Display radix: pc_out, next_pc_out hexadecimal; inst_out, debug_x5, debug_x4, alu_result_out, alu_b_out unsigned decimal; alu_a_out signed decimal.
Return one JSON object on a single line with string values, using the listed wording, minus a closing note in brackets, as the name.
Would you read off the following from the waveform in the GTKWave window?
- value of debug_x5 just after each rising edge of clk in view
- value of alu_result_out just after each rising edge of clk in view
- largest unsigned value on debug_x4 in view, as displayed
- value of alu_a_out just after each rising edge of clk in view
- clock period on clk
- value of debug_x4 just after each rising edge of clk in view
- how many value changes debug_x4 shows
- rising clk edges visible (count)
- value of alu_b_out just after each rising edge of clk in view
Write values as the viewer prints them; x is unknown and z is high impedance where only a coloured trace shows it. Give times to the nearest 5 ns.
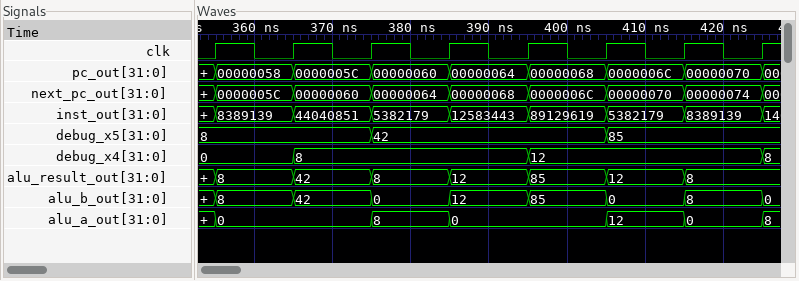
{"value of debug_x5 just after each rising edge of clk in view": "8, 8, 42, 42, 42, 85, 85, 85", "value of alu_result_out just after each rising edge of clk in view": "8, 42, 8, 12, 85, 12, 8, 8", "largest unsigned value on debug_x4 in view, as displayed": "12", "value of alu_a_out just after each rising edge of clk in view": "0, 0, 8, 0, 0, 12, 0, 8", "clock period on clk": "10 ns", "value of debug_x4 just after each rising edge of clk in view": "0, 8, 8, 8, 12, 12, 12, 8", "how many value changes debug_x4 shows": "3", "rising clk edges visible": "8", "value of alu_b_out just after each rising edge of clk in view": "8, 42, 0, 12, 85, 0, 8, 0"}
